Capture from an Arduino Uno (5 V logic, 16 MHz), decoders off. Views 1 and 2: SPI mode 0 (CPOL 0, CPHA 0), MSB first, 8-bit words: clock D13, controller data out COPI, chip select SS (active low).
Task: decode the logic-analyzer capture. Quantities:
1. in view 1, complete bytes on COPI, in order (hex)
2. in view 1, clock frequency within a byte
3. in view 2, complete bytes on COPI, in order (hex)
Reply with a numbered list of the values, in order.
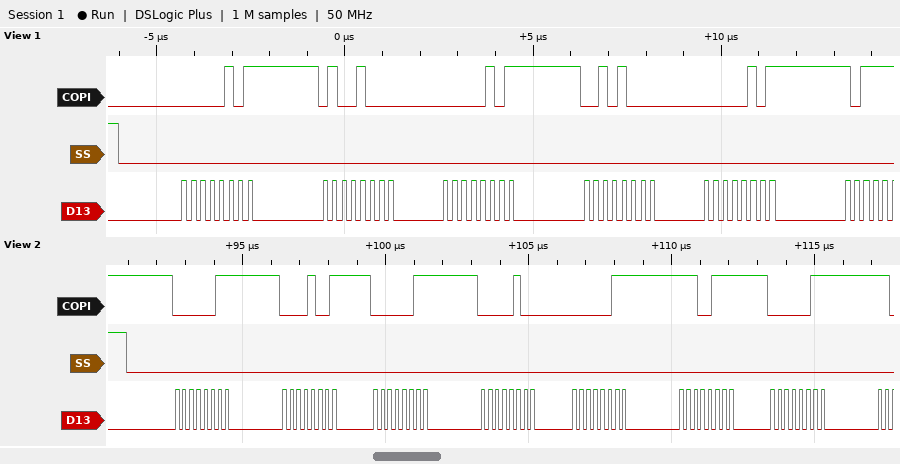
1. 05 48 05 28 05
2. 4 MHz
3. 03 09 03 04 03 E7 03
